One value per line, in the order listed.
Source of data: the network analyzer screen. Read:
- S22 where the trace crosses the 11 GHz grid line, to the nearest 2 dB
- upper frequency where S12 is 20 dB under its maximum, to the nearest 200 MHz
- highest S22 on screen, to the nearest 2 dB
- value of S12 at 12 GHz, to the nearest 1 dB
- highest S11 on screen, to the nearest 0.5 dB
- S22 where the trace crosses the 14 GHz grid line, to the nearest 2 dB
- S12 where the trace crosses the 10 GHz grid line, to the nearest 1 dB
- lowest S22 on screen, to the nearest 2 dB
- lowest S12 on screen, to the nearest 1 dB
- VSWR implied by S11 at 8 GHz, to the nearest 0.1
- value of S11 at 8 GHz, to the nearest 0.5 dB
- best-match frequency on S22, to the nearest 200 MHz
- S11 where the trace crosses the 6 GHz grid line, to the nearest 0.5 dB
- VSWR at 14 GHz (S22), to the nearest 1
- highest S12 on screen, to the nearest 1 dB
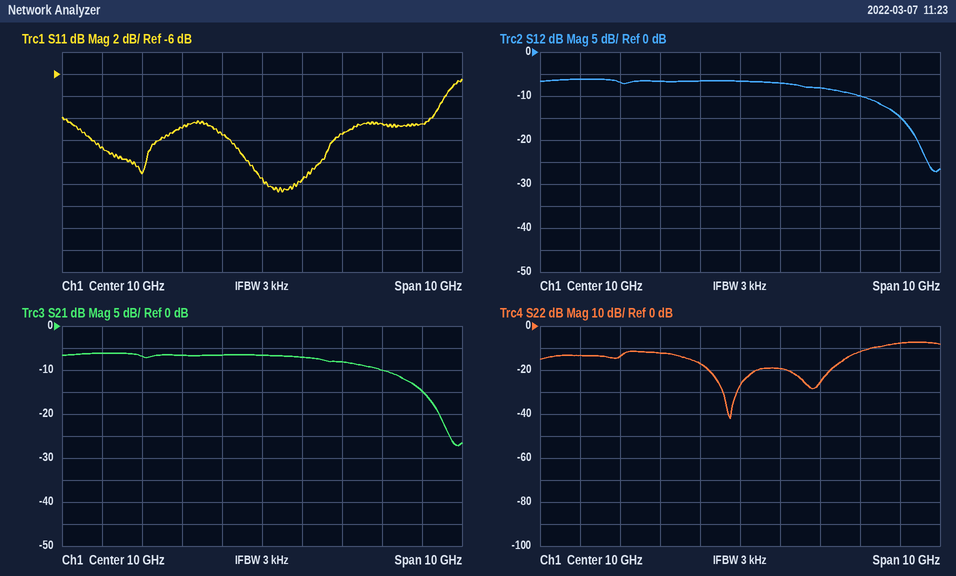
-20 dB
14.8 GHz
-8 dB
-8 dB
-6.5 dB
-8 dB
-7 dB
-42 dB
-27 dB
1.8
-11.0 dB
9.8 GHz
-12.5 dB
2
-6 dB
